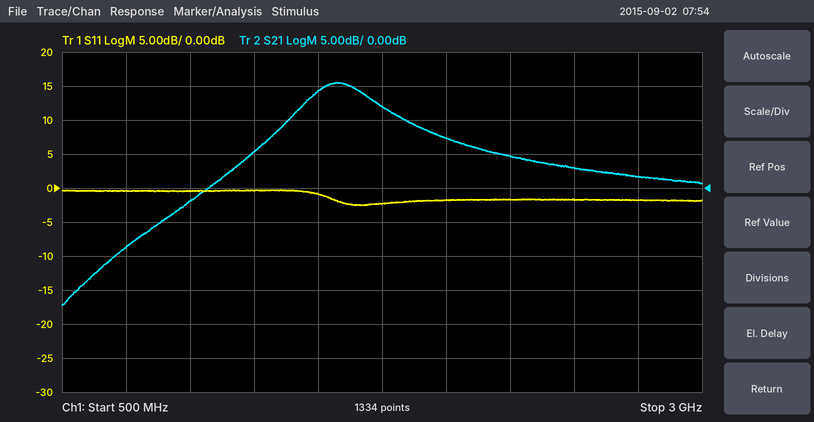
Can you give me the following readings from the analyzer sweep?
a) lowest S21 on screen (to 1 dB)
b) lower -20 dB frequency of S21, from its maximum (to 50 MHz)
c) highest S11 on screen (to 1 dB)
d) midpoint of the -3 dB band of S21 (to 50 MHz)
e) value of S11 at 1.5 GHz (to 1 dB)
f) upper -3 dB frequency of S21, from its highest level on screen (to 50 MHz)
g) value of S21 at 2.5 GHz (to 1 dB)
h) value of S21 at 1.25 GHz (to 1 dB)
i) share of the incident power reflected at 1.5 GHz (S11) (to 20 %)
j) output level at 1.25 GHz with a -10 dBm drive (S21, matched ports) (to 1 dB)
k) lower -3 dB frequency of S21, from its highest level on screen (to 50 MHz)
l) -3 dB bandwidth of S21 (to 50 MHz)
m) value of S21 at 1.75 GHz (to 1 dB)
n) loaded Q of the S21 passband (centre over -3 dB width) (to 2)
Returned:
-17 dB
900 MHz
0 dB
1.60 GHz
-1 dB
1.75 GHz
3 dB
5 dB
80 %
-5 dBm
1.45 GHz
300 MHz
12 dB
6
